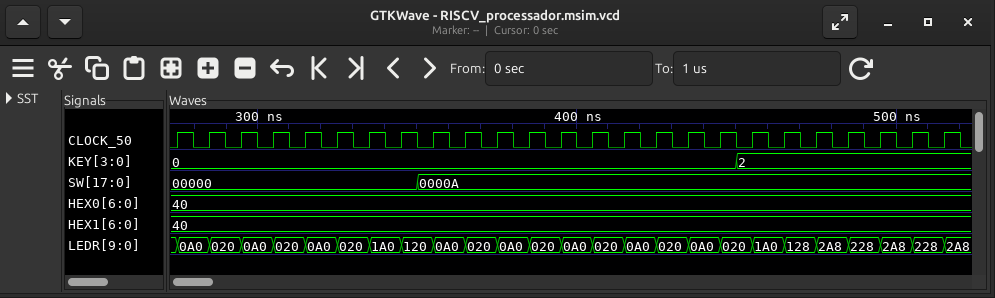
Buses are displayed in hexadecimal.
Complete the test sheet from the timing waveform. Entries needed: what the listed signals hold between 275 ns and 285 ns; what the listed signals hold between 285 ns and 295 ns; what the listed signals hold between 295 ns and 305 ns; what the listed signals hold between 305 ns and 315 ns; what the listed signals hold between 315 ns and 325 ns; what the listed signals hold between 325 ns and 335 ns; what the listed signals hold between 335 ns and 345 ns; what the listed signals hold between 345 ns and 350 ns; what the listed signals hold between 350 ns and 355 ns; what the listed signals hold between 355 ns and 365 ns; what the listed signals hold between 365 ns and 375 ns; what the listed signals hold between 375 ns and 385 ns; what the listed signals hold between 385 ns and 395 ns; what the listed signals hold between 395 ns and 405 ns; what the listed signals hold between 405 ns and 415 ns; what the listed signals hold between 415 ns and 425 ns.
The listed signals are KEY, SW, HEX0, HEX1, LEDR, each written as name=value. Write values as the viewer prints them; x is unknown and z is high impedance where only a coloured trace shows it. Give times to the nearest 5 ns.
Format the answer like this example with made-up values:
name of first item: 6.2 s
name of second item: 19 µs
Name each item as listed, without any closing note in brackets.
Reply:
what the listed signals hold between 275 ns and 285 ns: KEY=0, SW=00000, HEX0=40, HEX1=40, LEDR=0A0
what the listed signals hold between 285 ns and 295 ns: KEY=0, SW=00000, HEX0=40, HEX1=40, LEDR=020
what the listed signals hold between 295 ns and 305 ns: KEY=0, SW=00000, HEX0=40, HEX1=40, LEDR=0A0
what the listed signals hold between 305 ns and 315 ns: KEY=0, SW=00000, HEX0=40, HEX1=40, LEDR=020
what the listed signals hold between 315 ns and 325 ns: KEY=0, SW=00000, HEX0=40, HEX1=40, LEDR=0A0
what the listed signals hold between 325 ns and 335 ns: KEY=0, SW=00000, HEX0=40, HEX1=40, LEDR=020
what the listed signals hold between 335 ns and 345 ns: KEY=0, SW=00000, HEX0=40, HEX1=40, LEDR=1A0
what the listed signals hold between 345 ns and 350 ns: KEY=0, SW=00000, HEX0=40, HEX1=40, LEDR=120
what the listed signals hold between 350 ns and 355 ns: KEY=0, SW=0000A, HEX0=40, HEX1=40, LEDR=120
what the listed signals hold between 355 ns and 365 ns: KEY=0, SW=0000A, HEX0=40, HEX1=40, LEDR=0A0
what the listed signals hold between 365 ns and 375 ns: KEY=0, SW=0000A, HEX0=40, HEX1=40, LEDR=020
what the listed signals hold between 375 ns and 385 ns: KEY=0, SW=0000A, HEX0=40, HEX1=40, LEDR=0A0
what the listed signals hold between 385 ns and 395 ns: KEY=0, SW=0000A, HEX0=40, HEX1=40, LEDR=020
what the listed signals hold between 395 ns and 405 ns: KEY=0, SW=0000A, HEX0=40, HEX1=40, LEDR=0A0
what the listed signals hold between 405 ns and 415 ns: KEY=0, SW=0000A, HEX0=40, HEX1=40, LEDR=020
what the listed signals hold between 415 ns and 425 ns: KEY=0, SW=0000A, HEX0=40, HEX1=40, LEDR=0A0
